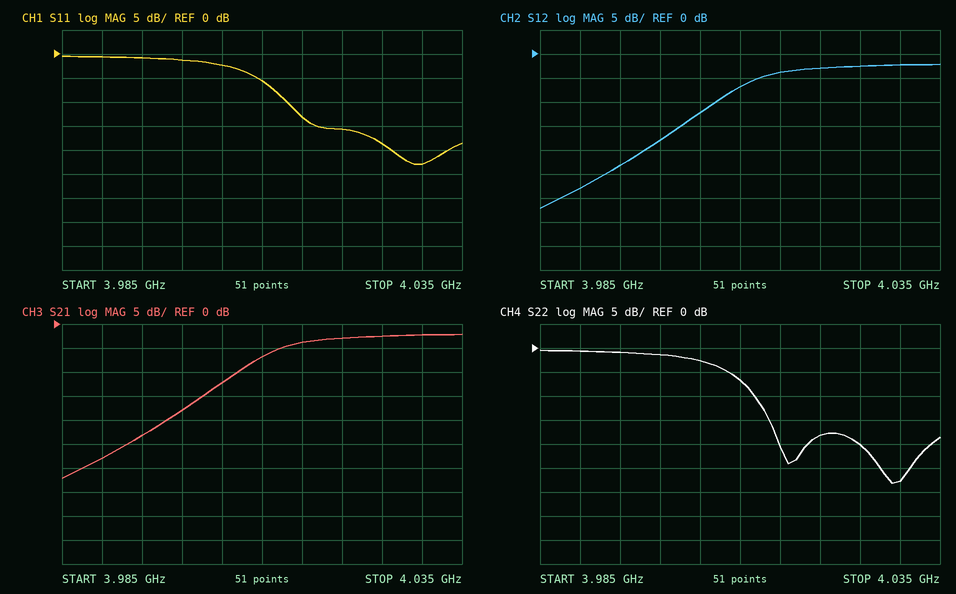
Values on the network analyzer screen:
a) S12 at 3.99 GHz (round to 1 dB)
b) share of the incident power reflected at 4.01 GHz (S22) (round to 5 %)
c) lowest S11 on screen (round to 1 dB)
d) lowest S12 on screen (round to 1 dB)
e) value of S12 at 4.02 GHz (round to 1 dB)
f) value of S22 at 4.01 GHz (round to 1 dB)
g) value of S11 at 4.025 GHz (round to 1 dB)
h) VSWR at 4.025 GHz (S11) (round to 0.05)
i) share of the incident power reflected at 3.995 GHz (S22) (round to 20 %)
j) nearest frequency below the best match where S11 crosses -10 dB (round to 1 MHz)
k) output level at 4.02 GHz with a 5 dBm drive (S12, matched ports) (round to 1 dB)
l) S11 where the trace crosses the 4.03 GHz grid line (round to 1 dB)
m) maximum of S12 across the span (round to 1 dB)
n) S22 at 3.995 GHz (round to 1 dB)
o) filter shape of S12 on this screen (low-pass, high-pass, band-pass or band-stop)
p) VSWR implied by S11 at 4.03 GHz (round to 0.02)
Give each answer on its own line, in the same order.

-28 dB
20 %
-23 dB
-32 dB
-3 dB
-7 dB
-19 dB
1.25
80 %
4.013 GHz
2 dBm
-23 dB
-2 dB
-1 dB
high-pass
1.16
